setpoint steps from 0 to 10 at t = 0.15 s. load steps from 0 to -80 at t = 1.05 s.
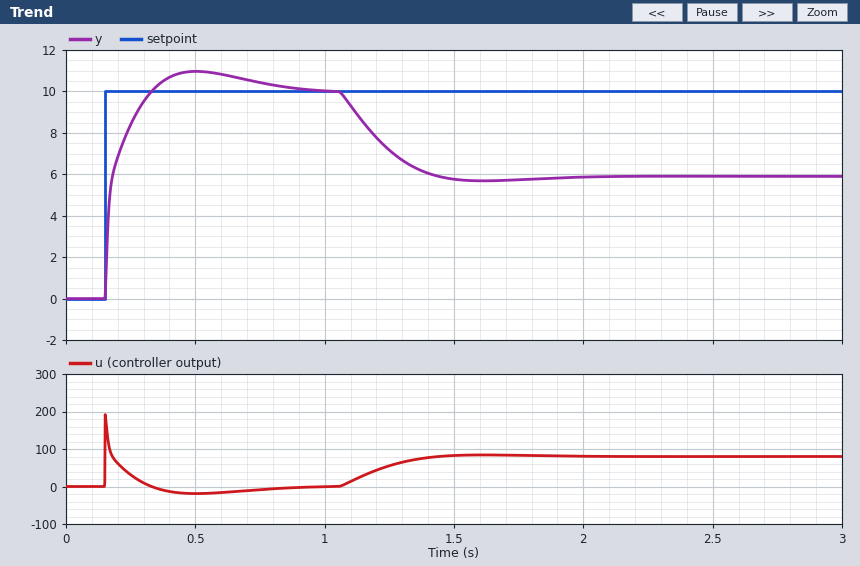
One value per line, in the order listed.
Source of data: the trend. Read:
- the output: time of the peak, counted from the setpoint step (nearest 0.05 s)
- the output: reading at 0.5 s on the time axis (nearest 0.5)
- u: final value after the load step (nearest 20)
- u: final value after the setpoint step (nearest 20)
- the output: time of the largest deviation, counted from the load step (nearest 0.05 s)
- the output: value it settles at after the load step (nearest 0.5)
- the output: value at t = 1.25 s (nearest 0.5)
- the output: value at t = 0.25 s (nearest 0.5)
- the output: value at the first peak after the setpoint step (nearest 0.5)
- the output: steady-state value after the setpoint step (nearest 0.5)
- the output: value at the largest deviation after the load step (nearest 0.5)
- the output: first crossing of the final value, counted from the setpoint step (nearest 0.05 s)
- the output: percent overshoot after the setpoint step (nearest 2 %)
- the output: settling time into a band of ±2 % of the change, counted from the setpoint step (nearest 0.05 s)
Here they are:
0.35 s
11.0
80
0
0.55 s
6.0
7.0
8.5
11.0
10.0
5.5
0.20 s
10 %
0.70 s
